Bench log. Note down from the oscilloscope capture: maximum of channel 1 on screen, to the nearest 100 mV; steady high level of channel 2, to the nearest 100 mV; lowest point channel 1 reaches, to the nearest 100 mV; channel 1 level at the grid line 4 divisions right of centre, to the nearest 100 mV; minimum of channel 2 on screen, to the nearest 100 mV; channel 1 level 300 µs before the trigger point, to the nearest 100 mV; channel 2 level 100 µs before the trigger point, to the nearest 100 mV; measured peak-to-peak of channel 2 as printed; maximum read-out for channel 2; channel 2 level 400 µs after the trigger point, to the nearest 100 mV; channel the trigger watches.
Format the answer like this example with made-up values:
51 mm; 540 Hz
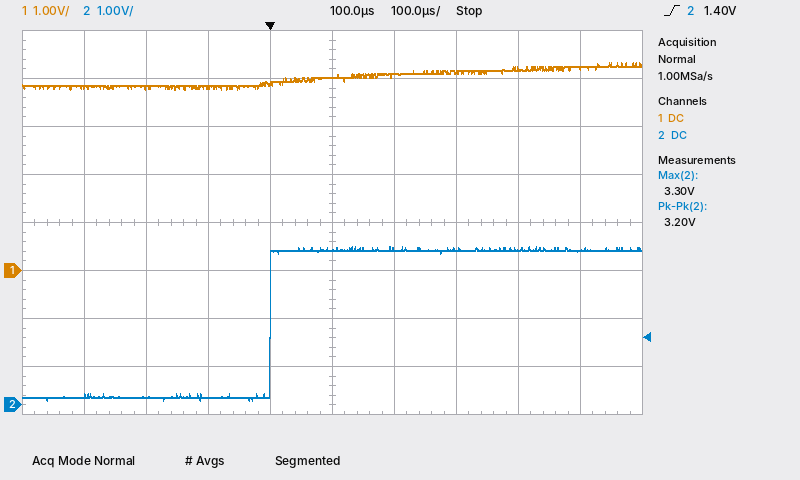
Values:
4.3 V; 3.2 V; 3.8 V; 4.2 V; 100 mV; 3.8 V; 200 mV; 3.20 V; 3.30 V; 3.2 V; channel 2
